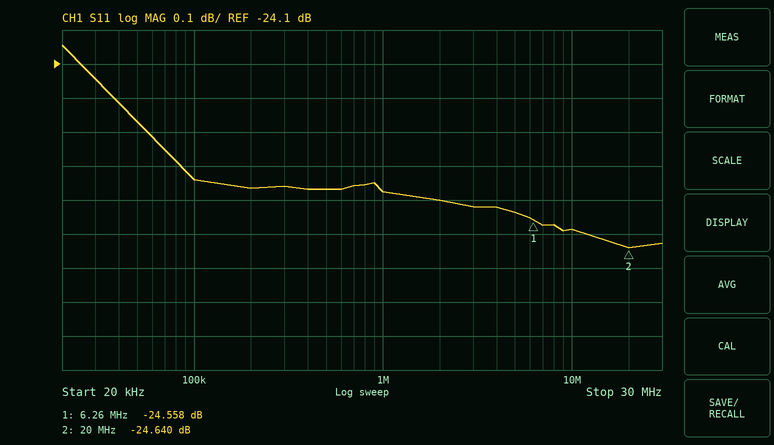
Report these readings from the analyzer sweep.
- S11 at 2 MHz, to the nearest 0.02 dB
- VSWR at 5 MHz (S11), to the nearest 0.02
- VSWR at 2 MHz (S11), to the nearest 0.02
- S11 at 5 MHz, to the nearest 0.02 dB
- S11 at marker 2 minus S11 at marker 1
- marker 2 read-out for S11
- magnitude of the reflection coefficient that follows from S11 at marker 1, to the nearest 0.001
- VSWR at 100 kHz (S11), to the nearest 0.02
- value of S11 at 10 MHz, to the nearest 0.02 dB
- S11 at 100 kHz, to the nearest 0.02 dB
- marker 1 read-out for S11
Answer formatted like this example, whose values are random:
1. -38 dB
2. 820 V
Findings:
1. -24.50 dB
2. 1.12
3. 1.12
4. -24.54 dB
5. -0.082 dB
6. -24.640 dB
7. 0.059
8. 1.12
9. -24.58 dB
10. -24.44 dB
11. -24.558 dB
